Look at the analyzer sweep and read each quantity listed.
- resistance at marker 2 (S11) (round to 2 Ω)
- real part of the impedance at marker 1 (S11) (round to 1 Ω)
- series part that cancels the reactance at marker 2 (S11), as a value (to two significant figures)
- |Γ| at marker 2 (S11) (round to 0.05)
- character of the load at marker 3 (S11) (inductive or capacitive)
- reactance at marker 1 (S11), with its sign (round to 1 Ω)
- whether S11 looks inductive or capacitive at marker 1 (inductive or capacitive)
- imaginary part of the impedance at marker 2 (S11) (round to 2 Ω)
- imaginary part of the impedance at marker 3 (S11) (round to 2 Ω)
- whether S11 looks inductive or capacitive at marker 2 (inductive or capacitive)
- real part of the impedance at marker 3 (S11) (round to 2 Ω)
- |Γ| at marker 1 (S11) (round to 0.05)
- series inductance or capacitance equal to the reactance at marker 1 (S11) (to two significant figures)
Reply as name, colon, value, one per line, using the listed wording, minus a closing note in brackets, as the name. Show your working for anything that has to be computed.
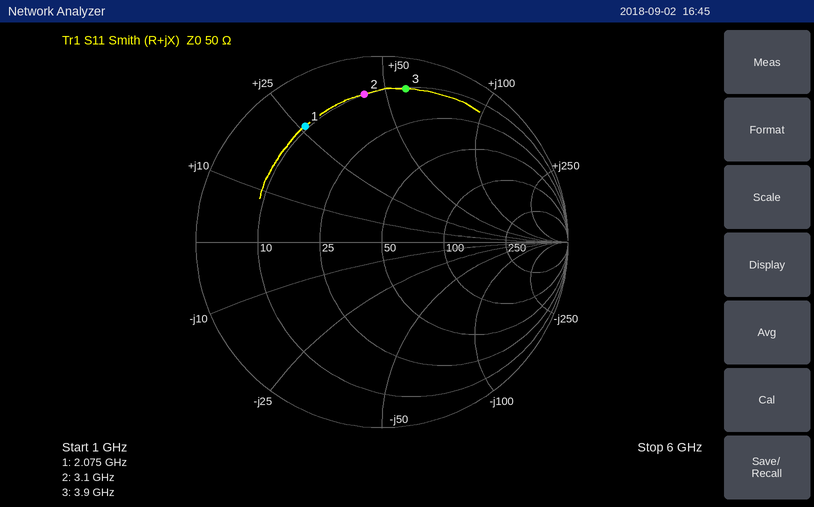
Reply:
resistance at marker 2 (S11): 10 Ω
real part of the impedance at marker 1 (S11): 9 Ω
series part that cancels the reactance at marker 2 (S11), as a value: C = 1/(2π × 3.1 GHz × 44 Ω) ≈ 1.2 pF
|Γ| at marker 2 (S11): 0.80
character of the load at marker 3 (S11): inductive
reactance at marker 1 (S11), with its sign: +26 Ω
whether S11 looks inductive or capacitive at marker 1: inductive
imaginary part of the impedance at marker 2 (S11): +44 Ω
imaginary part of the impedance at marker 3 (S11): +58 Ω
whether S11 looks inductive or capacitive at marker 2: inductive
real part of the impedance at marker 3 (S11): 10 Ω
|Γ| at marker 1 (S11): 0.75
series inductance or capacitance equal to the reactance at marker 1 (S11): L = 26 Ω/(2π × 2.075 GHz) ≈ 2.0 nH
